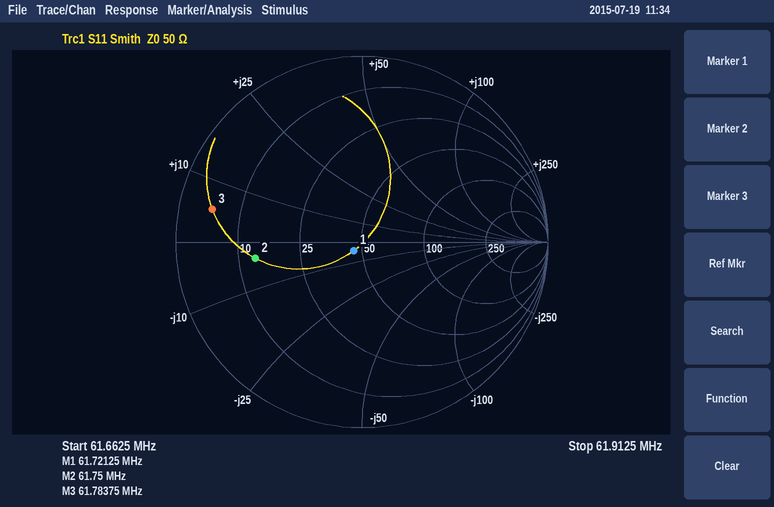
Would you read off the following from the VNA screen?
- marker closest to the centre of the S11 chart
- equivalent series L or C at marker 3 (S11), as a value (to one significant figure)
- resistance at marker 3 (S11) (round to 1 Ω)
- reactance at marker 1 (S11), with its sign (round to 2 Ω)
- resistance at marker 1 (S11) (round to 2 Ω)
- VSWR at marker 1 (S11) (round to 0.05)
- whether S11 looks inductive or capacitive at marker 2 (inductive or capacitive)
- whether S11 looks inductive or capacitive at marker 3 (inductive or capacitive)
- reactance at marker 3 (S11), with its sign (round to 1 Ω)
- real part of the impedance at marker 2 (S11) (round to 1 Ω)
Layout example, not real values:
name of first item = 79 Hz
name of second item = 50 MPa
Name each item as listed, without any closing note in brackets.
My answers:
marker closest to the centre of the S11 chart = marker 1
equivalent series L or C at marker 3 (S11), as a value = 10 nH
resistance at marker 3 (S11) = 5 Ω
reactance at marker 1 (S11), with its sign = -4 Ω
resistance at marker 1 (S11) = 46 Ω
VSWR at marker 1 (S11) = 1.15
whether S11 looks inductive or capacitive at marker 2 = capacitive
whether S11 looks inductive or capacitive at marker 3 = inductive
reactance at marker 3 (S11), with its sign = +5 Ω
real part of the impedance at marker 2 (S11) = 13 Ω
